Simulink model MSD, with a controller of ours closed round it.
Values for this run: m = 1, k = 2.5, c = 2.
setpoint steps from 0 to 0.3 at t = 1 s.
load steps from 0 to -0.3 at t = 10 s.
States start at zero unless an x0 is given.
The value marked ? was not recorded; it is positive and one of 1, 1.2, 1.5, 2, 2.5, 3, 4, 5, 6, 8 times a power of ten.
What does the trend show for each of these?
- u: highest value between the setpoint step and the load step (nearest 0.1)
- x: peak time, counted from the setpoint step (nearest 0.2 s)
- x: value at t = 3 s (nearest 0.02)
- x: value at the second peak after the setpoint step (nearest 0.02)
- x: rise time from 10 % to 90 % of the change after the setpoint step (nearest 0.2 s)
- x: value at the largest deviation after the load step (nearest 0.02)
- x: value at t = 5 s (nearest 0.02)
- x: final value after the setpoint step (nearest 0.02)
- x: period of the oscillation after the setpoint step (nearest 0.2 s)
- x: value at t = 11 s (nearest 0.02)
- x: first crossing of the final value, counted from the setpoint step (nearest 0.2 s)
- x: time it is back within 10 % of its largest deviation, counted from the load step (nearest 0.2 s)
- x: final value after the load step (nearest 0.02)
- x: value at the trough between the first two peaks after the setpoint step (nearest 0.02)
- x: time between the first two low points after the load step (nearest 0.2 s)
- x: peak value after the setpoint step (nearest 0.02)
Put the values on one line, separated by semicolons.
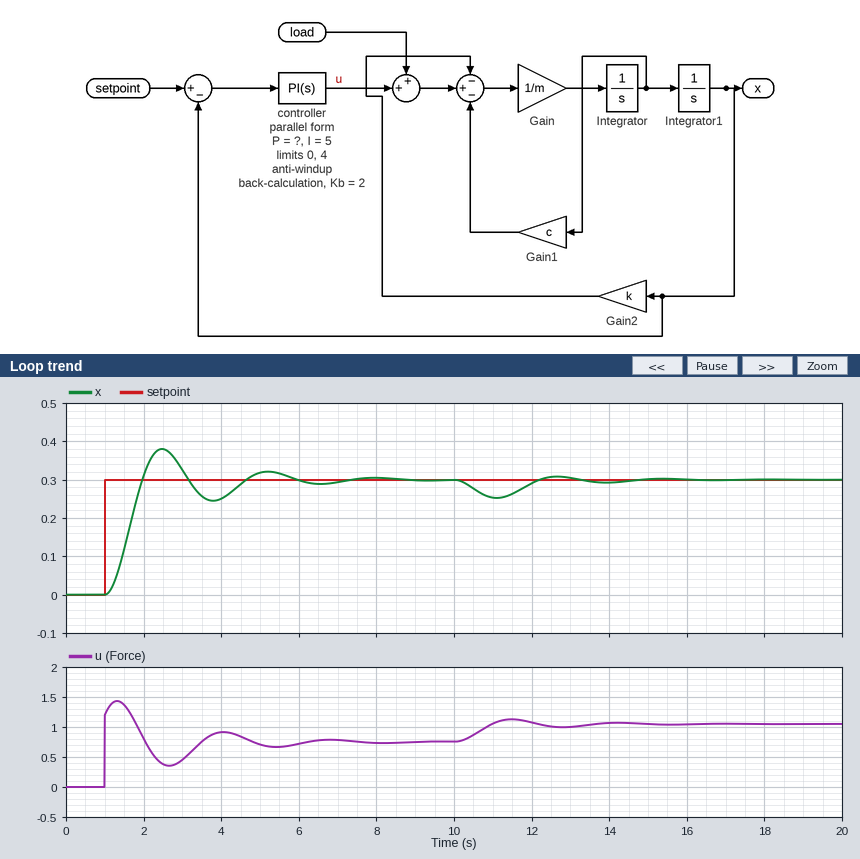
1.4; 1.4 s; 0.32; 0.32; 0.6 s; 0.26; 0.32; 0.30; 2.8 s; 0.26; 1.0 s; 4.4 s; 0.30; 0.24; 2.8 s; 0.38
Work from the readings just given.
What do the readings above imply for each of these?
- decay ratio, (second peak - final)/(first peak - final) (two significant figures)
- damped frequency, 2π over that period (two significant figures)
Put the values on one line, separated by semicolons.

0.25; 2.2 rad/s
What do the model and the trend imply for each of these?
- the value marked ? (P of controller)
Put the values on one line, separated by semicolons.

4
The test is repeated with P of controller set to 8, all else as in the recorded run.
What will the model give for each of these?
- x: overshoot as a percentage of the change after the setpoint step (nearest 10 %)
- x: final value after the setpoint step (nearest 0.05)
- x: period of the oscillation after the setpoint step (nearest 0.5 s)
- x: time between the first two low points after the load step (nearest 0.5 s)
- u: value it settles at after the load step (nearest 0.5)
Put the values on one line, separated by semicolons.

30 %; 0.30; 2.0 s; 2.0 s; 1.0
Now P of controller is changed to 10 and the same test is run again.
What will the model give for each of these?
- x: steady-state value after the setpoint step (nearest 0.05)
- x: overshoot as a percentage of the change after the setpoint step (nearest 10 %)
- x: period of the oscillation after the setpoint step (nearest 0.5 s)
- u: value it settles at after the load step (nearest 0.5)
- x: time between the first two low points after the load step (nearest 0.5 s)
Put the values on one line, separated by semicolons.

0.30; 30 %; 2.0 s; 1.0; 2.0 s
